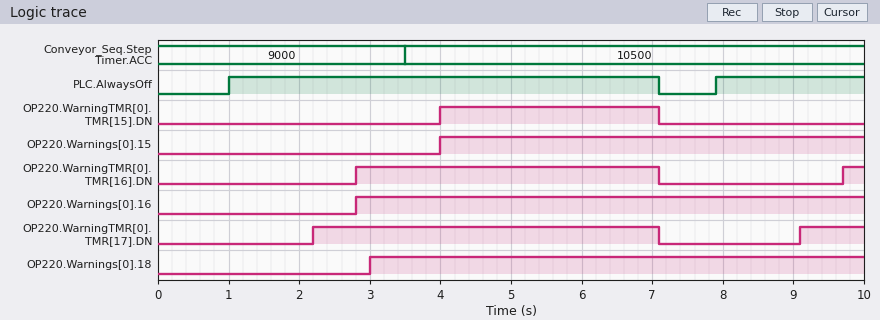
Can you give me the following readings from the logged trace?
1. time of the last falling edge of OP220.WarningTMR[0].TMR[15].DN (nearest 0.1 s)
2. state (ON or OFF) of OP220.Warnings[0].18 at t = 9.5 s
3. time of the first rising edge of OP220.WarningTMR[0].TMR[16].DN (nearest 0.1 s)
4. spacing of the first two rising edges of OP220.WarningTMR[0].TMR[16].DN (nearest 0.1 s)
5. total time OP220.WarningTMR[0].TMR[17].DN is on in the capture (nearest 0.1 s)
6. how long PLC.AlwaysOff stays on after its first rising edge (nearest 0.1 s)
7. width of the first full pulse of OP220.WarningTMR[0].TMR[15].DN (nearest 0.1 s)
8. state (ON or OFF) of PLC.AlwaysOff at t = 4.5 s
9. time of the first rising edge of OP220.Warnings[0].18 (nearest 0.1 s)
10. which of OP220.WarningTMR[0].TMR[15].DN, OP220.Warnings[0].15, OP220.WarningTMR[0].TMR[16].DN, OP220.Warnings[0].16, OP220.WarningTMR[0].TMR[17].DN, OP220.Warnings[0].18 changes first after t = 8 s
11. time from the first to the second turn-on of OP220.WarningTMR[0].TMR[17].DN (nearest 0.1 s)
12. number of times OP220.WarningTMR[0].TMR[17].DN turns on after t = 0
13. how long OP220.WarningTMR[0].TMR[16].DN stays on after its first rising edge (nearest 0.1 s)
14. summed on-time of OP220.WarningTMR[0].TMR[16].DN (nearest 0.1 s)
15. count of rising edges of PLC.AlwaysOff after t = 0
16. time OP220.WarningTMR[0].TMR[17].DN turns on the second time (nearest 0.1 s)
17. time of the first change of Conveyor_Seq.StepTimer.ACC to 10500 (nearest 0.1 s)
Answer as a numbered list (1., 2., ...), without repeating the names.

1. 7.1 s
2. ON
3. 2.8 s
4. 6.9 s
5. 5.8 s
6. 6.1 s
7. 3.1 s
8. ON
9. 3.0 s
10. OP220.WarningTMR[0].TMR[17].DN
11. 6.9 s
12. 2
13. 4.3 s
14. 4.6 s
15. 2
16. 9.1 s
17. 3.5 s
